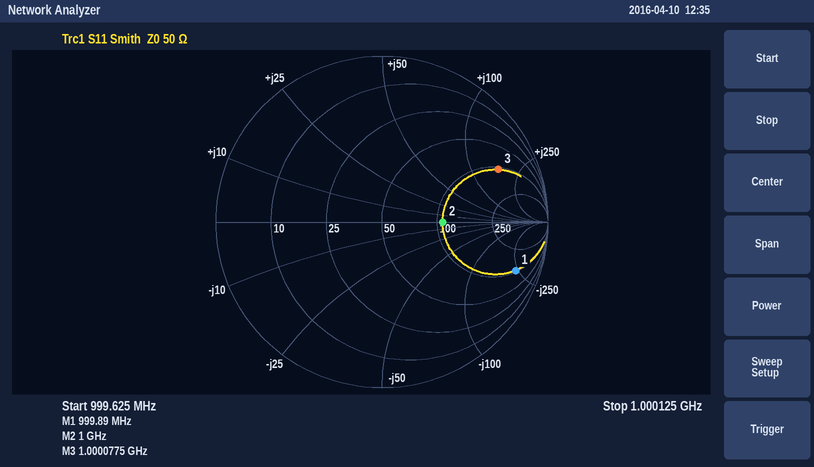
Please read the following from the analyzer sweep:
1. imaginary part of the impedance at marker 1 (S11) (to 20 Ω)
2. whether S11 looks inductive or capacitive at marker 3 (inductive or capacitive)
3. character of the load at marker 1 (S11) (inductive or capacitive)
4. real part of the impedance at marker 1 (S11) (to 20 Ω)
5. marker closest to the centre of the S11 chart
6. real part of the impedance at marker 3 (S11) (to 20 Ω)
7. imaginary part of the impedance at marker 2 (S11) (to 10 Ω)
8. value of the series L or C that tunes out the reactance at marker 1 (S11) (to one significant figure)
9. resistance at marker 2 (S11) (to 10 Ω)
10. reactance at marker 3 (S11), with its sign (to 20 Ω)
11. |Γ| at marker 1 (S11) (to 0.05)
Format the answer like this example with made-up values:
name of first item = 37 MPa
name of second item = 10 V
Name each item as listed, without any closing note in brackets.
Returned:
imaginary part of the impedance at marker 1 (S11) = -240 Ω
whether S11 looks inductive or capacitive at marker 3 = inductive
character of the load at marker 1 (S11) = capacitive
real part of the impedance at marker 1 (S11) = 100 Ω
marker closest to the centre of the S11 chart = marker 2
real part of the impedance at marker 3 (S11) = 100 Ω
imaginary part of the impedance at marker 2 (S11) = 0 Ω
value of the series L or C that tunes out the reactance at marker 1 (S11) = 40 nH
resistance at marker 2 (S11) = 110 Ω
reactance at marker 3 (S11), with its sign = +160 Ω
|Γ| at marker 1 (S11) = 0.85
